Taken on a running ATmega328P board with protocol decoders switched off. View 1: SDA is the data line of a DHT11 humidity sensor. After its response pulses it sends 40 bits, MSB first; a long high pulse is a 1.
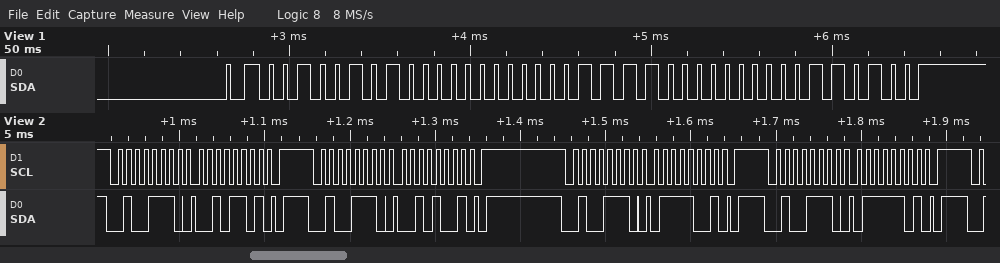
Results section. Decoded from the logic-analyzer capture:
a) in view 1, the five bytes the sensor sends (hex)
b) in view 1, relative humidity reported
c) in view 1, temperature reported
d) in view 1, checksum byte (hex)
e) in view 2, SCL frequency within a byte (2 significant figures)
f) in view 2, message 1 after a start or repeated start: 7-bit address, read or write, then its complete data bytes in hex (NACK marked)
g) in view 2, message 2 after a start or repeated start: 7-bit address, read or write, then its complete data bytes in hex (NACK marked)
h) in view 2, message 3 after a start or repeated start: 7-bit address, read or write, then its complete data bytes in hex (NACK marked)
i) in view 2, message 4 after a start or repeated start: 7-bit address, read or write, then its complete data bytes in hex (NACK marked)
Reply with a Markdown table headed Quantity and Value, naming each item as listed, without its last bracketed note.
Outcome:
| Quantity | Value |
|---|---|
| in view 1, the five bytes the sensor sends | 25 00 0F 00 34 |
| in view 1, relative humidity reported | 37 % |
| in view 1, temperature reported | 15.0 °C |
| in view 1, checksum byte | 0x34 |
| in view 2, SCL frequency within a byte | 100 kHz |
| in view 2, message 1 after a start or repeated start: 7-bit address, read or write, then its complete data bytes in hex | 0x27 write: 2D |
| in view 2, message 2 after a start or repeated start: 7-bit address, read or write, then its complete data bytes in hex | 0x27 write: 29 |
| in view 2, message 3 after a start or repeated start: 7-bit address, read or write, then its complete data bytes in hex | 0x27 write: 79 |
| in view 2, message 4 after a start or repeated start: 7-bit address, read or write, then its complete data bytes in hex | 0x27 write: 7D |
